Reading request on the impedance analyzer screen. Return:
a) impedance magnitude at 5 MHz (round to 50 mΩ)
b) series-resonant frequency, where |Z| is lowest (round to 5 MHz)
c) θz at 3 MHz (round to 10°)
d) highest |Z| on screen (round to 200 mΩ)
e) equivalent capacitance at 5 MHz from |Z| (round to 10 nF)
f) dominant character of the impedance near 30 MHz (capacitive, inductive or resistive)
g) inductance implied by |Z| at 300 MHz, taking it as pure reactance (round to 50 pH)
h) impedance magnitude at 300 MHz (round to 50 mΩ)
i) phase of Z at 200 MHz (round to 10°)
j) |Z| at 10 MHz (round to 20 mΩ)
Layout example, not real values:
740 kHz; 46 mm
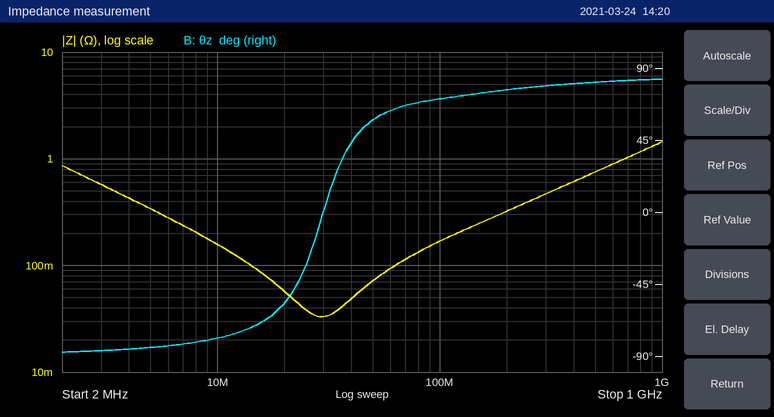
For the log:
350 mΩ; 30 MHz; -90°; 1.4 Ω; 90 nF; resistive; 250 pH; 450 mΩ; 80°; 160 mΩ
